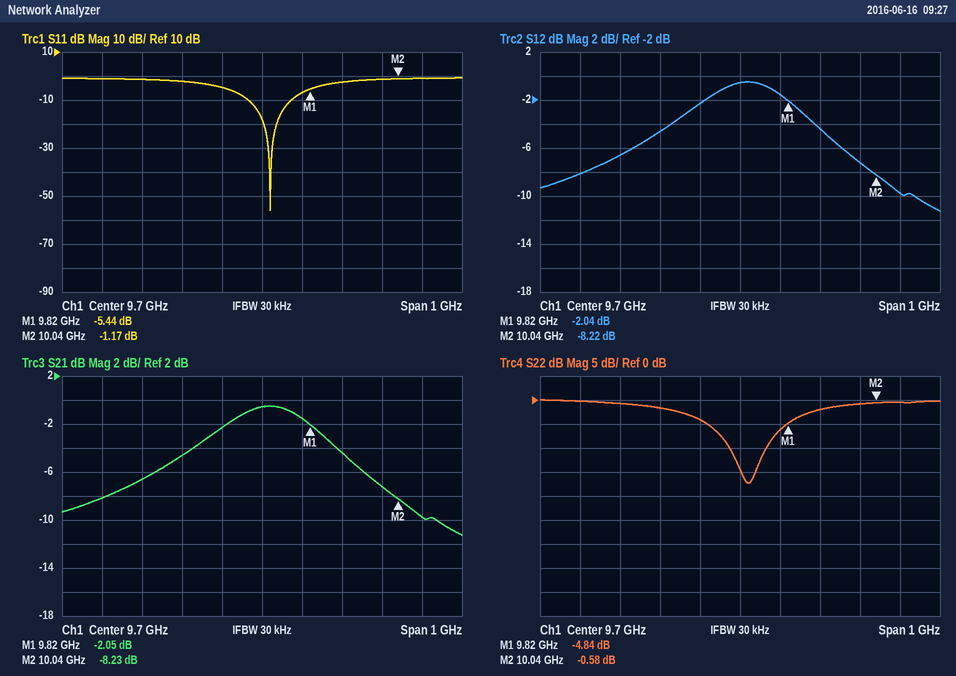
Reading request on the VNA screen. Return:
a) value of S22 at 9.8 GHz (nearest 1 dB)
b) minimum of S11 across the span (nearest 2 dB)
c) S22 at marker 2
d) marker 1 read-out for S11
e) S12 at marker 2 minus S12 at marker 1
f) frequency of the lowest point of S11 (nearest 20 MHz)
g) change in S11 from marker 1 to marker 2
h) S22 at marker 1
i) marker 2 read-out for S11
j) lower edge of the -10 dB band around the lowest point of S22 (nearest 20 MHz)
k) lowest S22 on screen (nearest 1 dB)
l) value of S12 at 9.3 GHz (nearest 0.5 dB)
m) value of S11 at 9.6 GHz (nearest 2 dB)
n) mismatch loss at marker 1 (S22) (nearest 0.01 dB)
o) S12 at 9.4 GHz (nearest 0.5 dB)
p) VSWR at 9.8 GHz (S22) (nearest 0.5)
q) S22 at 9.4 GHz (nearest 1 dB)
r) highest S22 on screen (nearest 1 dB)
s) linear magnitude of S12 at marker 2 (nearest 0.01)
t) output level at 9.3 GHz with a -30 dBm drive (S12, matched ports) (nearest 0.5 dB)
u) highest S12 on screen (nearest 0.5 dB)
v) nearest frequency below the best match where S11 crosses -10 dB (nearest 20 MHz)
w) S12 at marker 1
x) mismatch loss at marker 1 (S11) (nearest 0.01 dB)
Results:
-6 dB
-56 dB
-0.58 dB
-5.44 dB
-6.18 dB
9.72 GHz
4.27 dB
-4.84 dB
-1.17 dB
9.68 GHz
-17 dB
-8.0 dB
-4 dB
1.73 dB
-6.5 dB
3.0
-1 dB
0 dB
0.39
-38.0 dBm
-0.5 dB
9.66 GHz
-2.04 dB
1.46 dB
